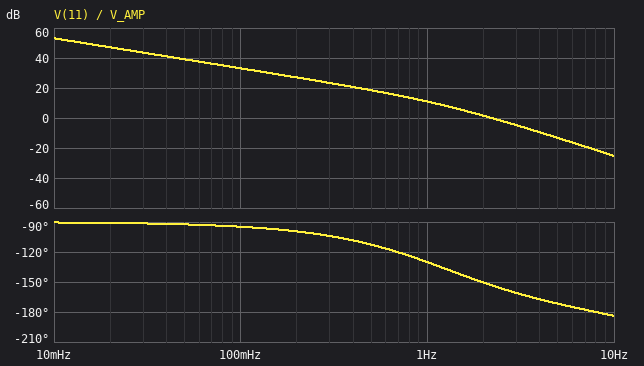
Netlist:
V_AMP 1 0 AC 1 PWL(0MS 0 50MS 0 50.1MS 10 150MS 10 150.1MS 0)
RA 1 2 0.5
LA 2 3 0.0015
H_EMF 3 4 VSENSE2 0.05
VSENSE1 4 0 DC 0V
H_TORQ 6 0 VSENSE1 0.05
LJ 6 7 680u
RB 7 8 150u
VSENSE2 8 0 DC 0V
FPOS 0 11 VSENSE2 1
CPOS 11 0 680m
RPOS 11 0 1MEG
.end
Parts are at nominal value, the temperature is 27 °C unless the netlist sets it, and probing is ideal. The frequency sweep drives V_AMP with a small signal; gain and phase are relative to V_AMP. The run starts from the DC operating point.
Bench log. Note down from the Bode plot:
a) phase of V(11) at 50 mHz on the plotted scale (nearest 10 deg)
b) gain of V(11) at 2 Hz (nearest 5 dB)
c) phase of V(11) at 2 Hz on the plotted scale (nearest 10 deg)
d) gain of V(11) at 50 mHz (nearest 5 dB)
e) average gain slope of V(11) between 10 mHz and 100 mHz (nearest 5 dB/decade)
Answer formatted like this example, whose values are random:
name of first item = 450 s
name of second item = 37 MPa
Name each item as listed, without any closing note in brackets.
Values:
phase of V(11) at 50 mHz on the plotted scale = -90 deg
gain of V(11) at 2 Hz = 0 dB
phase of V(11) at 2 Hz on the plotted scale = -150 deg
gain of V(11) at 50 mHz = 40 dB
average gain slope of V(11) between 10 mHz and 100 mHz = -20 dB/decade
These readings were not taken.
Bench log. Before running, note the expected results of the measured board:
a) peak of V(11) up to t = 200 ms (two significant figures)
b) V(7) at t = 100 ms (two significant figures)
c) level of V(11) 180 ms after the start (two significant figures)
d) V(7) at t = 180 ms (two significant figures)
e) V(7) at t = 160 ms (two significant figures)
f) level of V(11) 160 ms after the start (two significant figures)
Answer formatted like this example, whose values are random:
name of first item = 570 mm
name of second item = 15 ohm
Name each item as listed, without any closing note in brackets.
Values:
peak of V(11) up to t = 200 ms = 15 V
V(7) at t = 100 ms = 8.9 mV
level of V(11) 180 ms after the start = 12 V
V(7) at t = 180 ms = 13 mV
V(7) at t = 160 ms = 15 mV
level of V(11) 160 ms after the start = 9.7 V
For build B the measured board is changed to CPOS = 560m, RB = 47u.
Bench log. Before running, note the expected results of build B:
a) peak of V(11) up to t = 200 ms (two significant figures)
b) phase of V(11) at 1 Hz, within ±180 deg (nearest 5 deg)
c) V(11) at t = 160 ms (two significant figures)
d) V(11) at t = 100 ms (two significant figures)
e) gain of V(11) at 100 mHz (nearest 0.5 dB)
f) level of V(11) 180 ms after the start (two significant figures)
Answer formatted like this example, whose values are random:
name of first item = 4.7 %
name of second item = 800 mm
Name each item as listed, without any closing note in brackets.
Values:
peak of V(11) up to t = 200 ms = 18 V
phase of V(11) at 1 Hz, within ±180 deg = -130 deg
V(11) at t = 160 ms = 12 V
V(11) at t = 100 ms = 2.6 V
gain of V(11) at 100 mHz = 35.0 dB
level of V(11) 180 ms after the start = 15 V
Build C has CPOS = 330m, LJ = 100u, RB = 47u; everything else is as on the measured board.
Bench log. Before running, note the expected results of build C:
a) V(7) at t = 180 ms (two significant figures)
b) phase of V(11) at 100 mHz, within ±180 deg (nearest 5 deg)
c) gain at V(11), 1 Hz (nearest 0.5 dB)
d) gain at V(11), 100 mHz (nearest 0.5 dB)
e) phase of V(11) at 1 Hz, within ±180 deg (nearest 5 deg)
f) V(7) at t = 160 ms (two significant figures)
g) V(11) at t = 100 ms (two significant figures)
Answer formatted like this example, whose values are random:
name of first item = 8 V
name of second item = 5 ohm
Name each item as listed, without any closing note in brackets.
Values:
V(7) at t = 180 ms = 1.9 mV
phase of V(11) at 100 mHz, within ±180 deg = -90 deg
gain at V(11), 1 Hz = 19.5 dB
gain at V(11), 100 mHz = 39.5 dB
phase of V(11) at 1 Hz, within ±180 deg = -95 deg
V(7) at t = 160 ms = 6.3 mV
V(11) at t = 100 ms = 19 V
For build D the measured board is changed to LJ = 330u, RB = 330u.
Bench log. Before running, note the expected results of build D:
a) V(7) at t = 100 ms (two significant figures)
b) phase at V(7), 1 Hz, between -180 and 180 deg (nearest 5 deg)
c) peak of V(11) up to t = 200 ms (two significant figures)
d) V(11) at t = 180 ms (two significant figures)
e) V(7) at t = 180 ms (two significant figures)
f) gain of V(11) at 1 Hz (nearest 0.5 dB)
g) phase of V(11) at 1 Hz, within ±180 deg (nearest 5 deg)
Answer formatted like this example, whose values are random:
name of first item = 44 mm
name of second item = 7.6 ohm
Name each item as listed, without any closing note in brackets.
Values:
V(7) at t = 100 ms = 34 mV
phase at V(7), 1 Hz, between -180 and 180 deg = -20 deg
peak of V(11) up to t = 200 ms = 22 V
V(11) at t = 180 ms = 19 V
V(7) at t = 180 ms = 32 mV
gain of V(11) at 1 Hz = 12.5 dB
phase of V(11) at 1 Hz, within ±180 deg = -110 deg
